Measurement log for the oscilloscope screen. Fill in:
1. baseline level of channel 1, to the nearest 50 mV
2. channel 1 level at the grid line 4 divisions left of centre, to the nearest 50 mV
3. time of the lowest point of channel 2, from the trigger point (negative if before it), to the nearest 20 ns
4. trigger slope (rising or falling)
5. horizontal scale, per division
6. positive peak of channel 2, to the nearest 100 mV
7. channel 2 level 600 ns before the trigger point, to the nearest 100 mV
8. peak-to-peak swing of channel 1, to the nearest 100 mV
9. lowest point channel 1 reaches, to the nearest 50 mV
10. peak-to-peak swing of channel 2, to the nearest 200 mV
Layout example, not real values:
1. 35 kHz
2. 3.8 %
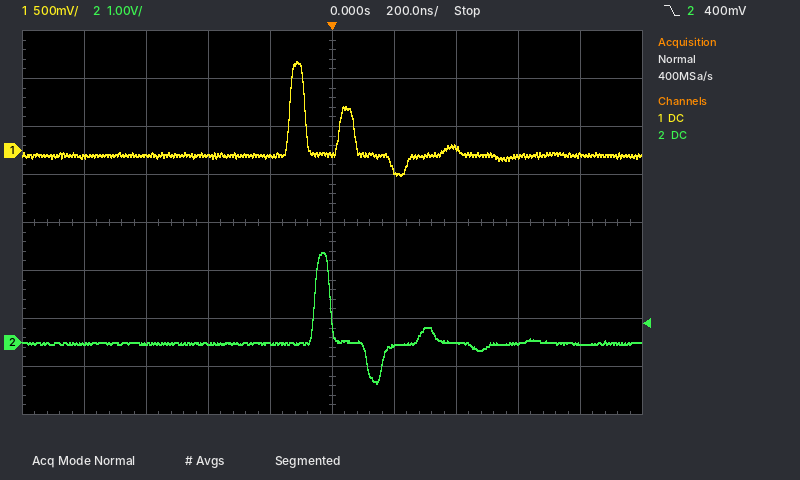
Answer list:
1. -50 mV
2. -50 mV
3. +140 ns
4. falling
5. 200 ns
6. 1.9 V
7. 0.0 V
8. 1.20 V
9. -250 mV
10. 2.8 V
